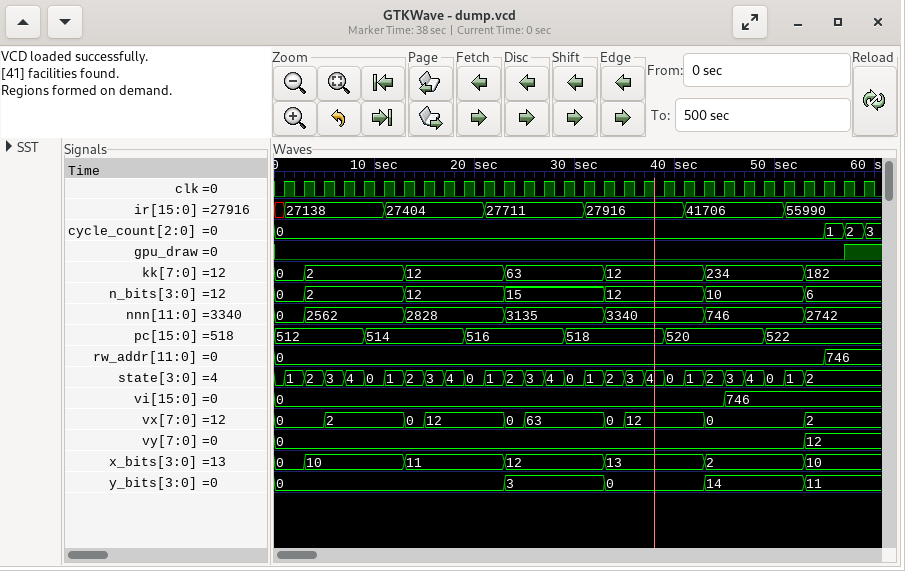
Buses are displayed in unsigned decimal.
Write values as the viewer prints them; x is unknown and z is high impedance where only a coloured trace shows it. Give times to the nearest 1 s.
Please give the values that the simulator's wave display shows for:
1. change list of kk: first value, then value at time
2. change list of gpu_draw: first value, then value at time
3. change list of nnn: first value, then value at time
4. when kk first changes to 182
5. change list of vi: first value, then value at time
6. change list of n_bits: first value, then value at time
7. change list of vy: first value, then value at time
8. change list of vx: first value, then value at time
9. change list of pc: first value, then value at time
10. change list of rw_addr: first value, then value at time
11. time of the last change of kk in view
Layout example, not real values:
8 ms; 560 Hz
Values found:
0, 2 at 3 s, 12 at 13 s, 63 at 23 s, 12 at 33 s, 234 at 43 s, 182 at 53 s; 0, 1 at 57 s; 0, 2562 at 3 s, 2828 at 13 s, 3135 at 23 s, 3340 at 33 s, 746 at 43 s, 2742 at 53 s; 53 s; 0, 746 at 45 s; 0, 2 at 3 s, 12 at 13 s, 15 at 23 s, 12 at 33 s, 10 at 43 s, 6 at 53 s; 0, 12 at 53 s; 0, 2 at 5 s, 0 at 13 s, 12 at 15 s, 0 at 23 s, 63 at 25 s, 0 at 33 s, 12 at 35 s, 0 at 43 s, 2 at 53 s; 512, 514 at 9 s, 516 at 19 s, 518 at 29 s, 520 at 39 s, 522 at 49 s; 0, 746 at 55 s; 53 s
